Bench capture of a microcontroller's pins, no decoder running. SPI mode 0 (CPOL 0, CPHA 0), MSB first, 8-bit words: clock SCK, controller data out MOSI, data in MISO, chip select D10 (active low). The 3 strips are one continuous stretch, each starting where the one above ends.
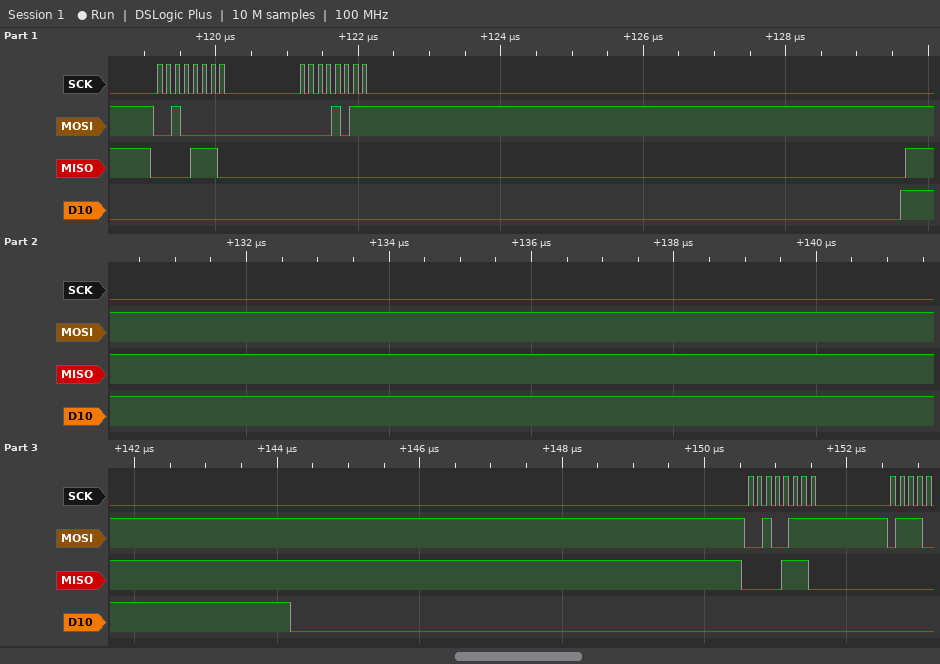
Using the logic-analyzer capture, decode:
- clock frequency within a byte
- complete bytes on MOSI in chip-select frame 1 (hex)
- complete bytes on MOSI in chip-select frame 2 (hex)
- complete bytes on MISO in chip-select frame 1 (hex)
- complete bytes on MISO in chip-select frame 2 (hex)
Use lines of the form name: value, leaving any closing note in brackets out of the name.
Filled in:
clock frequency within a byte: 8 MHz
complete bytes on MOSI in chip-select frame 1: 0x20 0x0B
complete bytes on MOSI in chip-select frame 2: 0x27
complete bytes on MISO in chip-select frame 1: 0x0E 0x00
complete bytes on MISO in chip-select frame 2: 0x0E
